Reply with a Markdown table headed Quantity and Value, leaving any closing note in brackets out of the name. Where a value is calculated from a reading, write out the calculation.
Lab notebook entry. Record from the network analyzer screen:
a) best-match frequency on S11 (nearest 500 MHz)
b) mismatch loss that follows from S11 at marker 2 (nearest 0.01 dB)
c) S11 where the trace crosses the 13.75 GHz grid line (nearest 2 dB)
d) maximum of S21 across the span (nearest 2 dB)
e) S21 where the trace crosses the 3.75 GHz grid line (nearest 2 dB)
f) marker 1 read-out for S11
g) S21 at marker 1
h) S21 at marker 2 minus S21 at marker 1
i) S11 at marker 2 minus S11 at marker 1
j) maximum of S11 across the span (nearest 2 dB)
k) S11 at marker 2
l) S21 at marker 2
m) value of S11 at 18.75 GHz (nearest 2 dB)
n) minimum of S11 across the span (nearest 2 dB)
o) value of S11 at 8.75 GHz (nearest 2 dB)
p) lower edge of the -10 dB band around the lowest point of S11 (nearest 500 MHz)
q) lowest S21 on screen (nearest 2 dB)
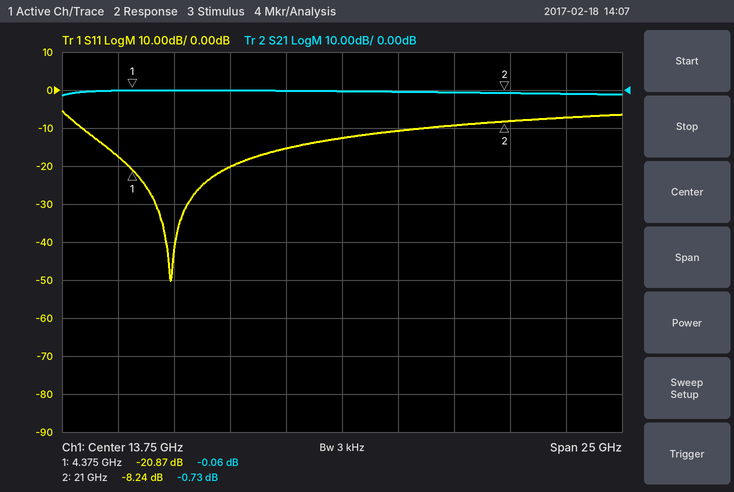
| Quantity | Value |
|---|---|
| best-match frequency on S11 | 6.0 GHz |
| mismatch loss that follows from S11 at marker 2 | −10 log10(1 − 10^(-8.24/10)) ≈ 0.71 dB |
| S11 where the trace crosses the 13.75 GHz grid line | -12 dB |
| maximum of S21 across the span | 0 dB |
| S21 where the trace crosses the 3.75 GHz grid line | 0 dB |
| marker 1 read-out for S11 | -20.87 dB |
| S21 at marker 1 | -0.06 dB |
| S21 at marker 2 minus S21 at marker 1 | -0.73 − (-0.06) = -0.67 dB |
| S11 at marker 2 minus S11 at marker 1 | -8.24 − (-20.87) = 12.63 dB |
| maximum of S11 across the span | -6 dB |
| S11 at marker 2 | -8.24 dB |
| S21 at marker 2 | -0.73 dB |
| value of S11 at 18.75 GHz | -10 dB |
| minimum of S11 across the span | -50 dB |
| value of S11 at 8.75 GHz | -20 dB |
| lower edge of the -10 dB band around the lowest point of S11 | 2.0 GHz |
| lowest S21 on screen | -2 dB |
